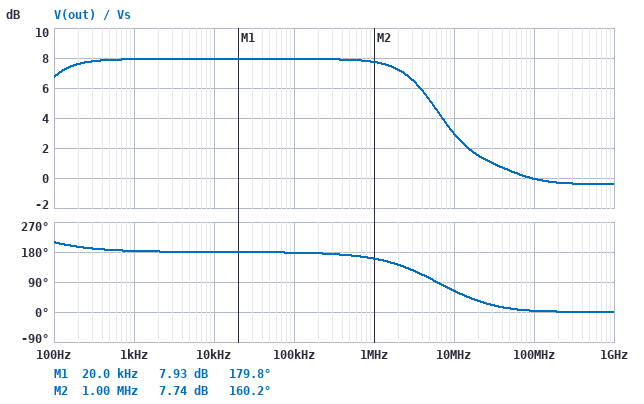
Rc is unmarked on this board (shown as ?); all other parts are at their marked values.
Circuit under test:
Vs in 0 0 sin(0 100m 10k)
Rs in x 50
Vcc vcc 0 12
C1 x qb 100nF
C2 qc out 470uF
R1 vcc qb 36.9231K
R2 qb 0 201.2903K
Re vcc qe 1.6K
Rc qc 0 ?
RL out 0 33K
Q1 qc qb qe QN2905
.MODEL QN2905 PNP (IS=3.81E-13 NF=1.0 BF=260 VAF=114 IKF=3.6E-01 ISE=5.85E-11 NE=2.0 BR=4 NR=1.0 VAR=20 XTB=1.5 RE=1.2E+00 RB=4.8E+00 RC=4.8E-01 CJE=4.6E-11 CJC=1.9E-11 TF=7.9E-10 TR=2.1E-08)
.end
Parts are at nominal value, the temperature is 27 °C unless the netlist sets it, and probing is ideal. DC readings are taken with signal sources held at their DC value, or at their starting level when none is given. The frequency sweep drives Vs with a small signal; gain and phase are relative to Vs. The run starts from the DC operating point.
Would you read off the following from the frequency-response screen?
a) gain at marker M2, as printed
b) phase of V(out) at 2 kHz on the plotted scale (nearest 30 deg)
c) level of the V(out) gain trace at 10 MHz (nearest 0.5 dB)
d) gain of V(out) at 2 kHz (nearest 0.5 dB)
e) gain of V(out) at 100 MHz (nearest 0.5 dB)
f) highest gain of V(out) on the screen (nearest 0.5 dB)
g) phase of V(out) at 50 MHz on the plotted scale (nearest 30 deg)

7.74 dB
180 deg
3.0 dB
8.0 dB
0 dB
8.0 dB
0 deg
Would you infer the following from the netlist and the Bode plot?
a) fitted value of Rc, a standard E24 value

4.7 kΩ
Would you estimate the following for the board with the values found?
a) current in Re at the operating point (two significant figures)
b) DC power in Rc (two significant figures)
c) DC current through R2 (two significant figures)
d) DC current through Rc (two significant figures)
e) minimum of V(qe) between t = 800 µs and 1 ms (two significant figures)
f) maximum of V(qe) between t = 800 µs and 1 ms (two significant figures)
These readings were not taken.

720 µA
2.4 mW
51 µA
710 µA
11 V
11 V
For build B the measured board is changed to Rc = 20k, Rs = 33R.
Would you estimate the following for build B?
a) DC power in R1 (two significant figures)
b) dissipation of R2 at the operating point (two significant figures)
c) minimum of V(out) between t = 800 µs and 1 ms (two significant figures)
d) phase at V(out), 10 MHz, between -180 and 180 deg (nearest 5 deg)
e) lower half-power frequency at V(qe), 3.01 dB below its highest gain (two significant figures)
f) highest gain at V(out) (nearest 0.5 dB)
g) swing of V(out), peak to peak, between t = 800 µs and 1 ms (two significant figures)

57 µW
550 µW
-940 mV
10 deg
1.1 kHz
0 dB
940 mV
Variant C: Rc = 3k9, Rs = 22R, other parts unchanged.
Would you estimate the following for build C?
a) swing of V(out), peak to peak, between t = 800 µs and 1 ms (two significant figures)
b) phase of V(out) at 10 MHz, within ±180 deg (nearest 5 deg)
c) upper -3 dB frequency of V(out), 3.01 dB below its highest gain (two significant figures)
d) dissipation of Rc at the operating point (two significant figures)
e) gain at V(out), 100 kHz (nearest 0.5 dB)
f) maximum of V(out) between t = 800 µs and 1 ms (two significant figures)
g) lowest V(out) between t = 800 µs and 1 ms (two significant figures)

420 mV
70 deg
8.0 MHz
2.0 mW
6.5 dB
210 mV
-210 mV
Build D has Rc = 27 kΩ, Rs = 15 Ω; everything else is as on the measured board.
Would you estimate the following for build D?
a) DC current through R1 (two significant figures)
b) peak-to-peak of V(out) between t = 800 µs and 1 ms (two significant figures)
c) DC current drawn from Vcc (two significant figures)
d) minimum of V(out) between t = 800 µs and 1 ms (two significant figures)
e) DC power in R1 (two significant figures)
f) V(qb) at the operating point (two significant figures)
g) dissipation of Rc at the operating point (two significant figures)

34 µA
870 mV
470 µA
-870 mV
42 µW
11 V
4.7 mW
